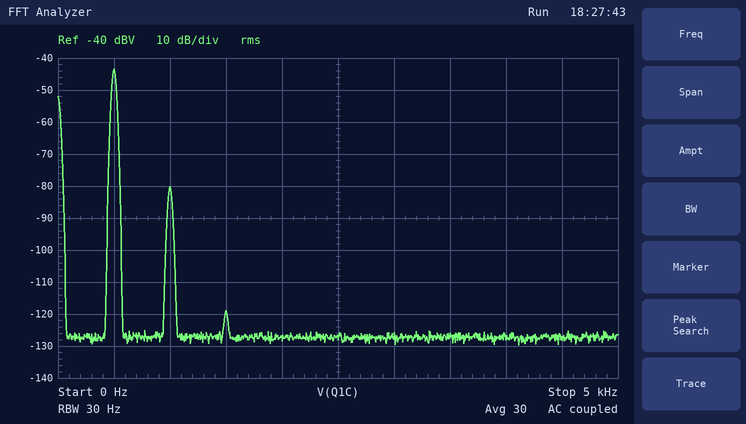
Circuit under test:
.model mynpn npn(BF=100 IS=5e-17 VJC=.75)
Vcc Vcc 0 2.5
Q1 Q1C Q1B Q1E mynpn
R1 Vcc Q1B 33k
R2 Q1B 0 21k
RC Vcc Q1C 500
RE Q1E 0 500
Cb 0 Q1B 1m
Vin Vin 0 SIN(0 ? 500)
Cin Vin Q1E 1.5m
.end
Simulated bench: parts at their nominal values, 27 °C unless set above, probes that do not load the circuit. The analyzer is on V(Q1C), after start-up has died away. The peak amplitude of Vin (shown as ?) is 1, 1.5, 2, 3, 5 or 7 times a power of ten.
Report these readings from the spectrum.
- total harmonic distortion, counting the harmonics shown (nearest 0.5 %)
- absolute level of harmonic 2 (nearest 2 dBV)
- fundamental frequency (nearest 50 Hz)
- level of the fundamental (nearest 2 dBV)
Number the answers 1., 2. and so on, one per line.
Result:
1. 1.5 %
2. -80 dBV
3. 500 Hz
4. -44 dBV
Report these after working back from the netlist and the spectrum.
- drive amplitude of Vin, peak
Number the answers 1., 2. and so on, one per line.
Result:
1. 1.5 mV
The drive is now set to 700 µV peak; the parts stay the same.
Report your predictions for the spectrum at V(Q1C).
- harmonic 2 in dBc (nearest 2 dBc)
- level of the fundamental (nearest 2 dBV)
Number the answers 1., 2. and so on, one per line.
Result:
1. -44 dBc
2. -50 dBV
